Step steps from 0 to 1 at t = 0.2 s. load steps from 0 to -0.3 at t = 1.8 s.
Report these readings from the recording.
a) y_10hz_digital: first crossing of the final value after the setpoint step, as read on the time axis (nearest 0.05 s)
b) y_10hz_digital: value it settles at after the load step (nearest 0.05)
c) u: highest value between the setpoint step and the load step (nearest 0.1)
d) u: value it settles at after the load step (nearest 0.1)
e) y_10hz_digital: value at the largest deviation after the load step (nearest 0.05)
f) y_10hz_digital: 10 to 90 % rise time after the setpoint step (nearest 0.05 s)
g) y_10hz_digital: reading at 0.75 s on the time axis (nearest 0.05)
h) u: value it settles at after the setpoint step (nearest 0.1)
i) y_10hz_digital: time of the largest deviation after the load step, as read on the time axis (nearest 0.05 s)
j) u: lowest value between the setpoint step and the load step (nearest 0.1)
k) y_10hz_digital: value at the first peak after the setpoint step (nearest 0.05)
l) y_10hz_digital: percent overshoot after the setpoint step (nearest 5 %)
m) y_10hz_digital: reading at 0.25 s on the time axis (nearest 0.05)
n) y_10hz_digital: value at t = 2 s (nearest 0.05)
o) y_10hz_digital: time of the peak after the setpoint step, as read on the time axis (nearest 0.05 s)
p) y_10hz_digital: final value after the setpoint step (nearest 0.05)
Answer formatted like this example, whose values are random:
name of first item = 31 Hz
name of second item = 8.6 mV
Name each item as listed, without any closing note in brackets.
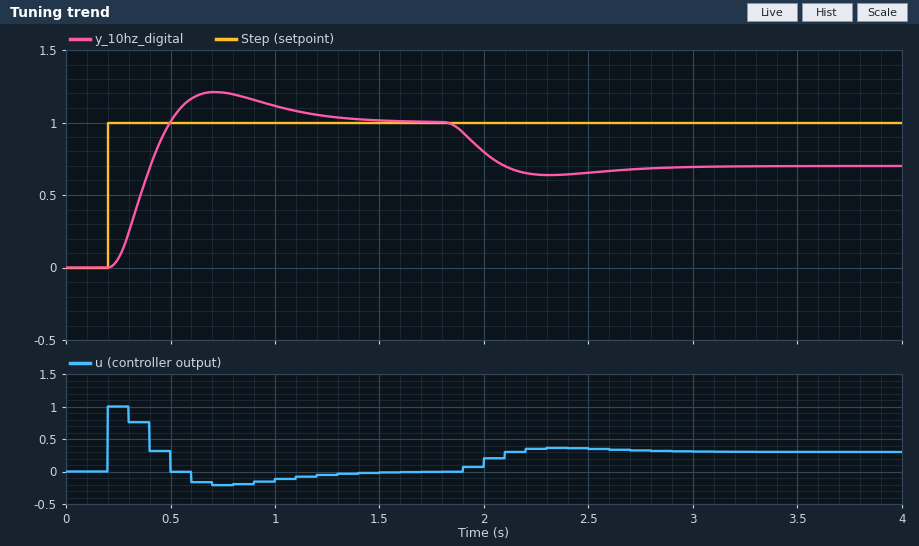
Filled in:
y_10hz_digital: first crossing of the final value after the setpoint step, as read on the time axis = 0.50 s
y_10hz_digital: value it settles at after the load step = 0.70
u: highest value between the setpoint step and the load step = 1.0
u: value it settles at after the load step = 0.3
y_10hz_digital: value at the largest deviation after the load step = 0.65
y_10hz_digital: 10 to 90 % rise time after the setpoint step = 0.20 s
y_10hz_digital: reading at 0.75 s on the time axis = 1.20
u: value it settles at after the setpoint step = 0.0
y_10hz_digital: time of the largest deviation after the load step, as read on the time axis = 2.30 s
u: lowest value between the setpoint step and the load step = -0.2
y_10hz_digital: value at the first peak after the setpoint step = 1.20
y_10hz_digital: percent overshoot after the setpoint step = 20 %
y_10hz_digital: reading at 0.25 s on the time axis = 0.05
y_10hz_digital: value at t = 2 s = 0.80
y_10hz_digital: time of the peak after the setpoint step, as read on the time axis = 0.70 s
y_10hz_digital: final value after the setpoint step = 1.00
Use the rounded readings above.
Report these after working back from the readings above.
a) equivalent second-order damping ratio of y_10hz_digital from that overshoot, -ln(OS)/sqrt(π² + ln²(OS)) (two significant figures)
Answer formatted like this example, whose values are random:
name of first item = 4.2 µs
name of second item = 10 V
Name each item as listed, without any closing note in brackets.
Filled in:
equivalent second-order damping ratio of y_10hz_digital from that overshoot, -ln(OS)/sqrt(π² + ln²(OS)) = 0.46
